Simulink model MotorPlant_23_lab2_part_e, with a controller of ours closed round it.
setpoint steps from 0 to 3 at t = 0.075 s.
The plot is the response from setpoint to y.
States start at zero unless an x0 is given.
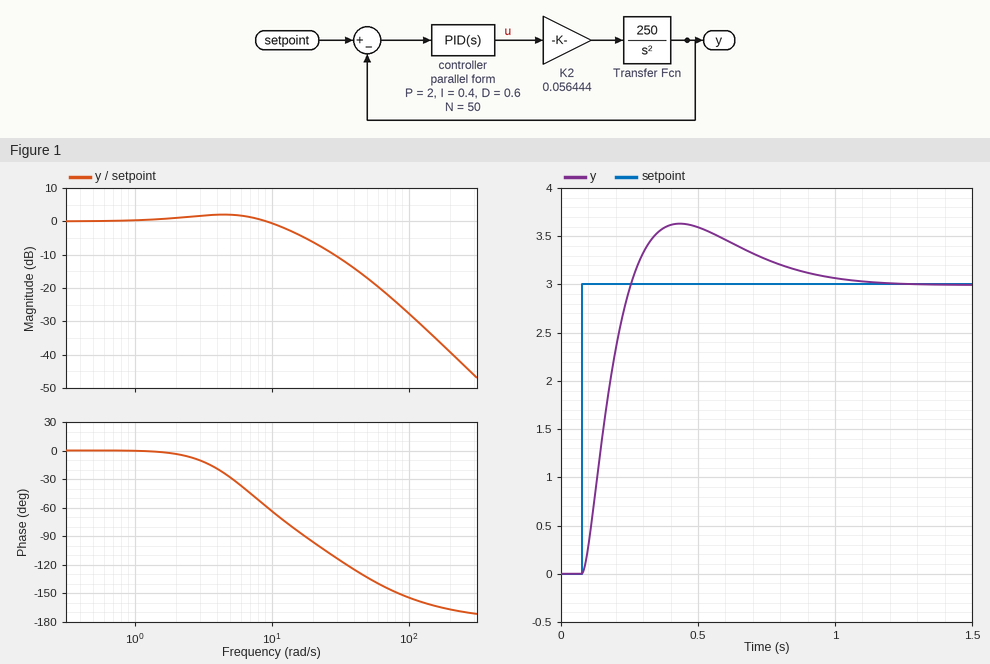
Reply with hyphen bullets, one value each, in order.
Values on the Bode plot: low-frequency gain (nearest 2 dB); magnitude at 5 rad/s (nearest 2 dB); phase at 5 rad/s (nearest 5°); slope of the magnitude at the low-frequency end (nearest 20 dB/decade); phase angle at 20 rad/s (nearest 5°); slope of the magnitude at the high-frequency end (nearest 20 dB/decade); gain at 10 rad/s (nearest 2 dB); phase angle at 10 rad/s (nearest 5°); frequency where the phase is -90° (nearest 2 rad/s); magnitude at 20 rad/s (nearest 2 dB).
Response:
- 0 dB
- 2 dB
- -30°
- 0 dB/decade
- -95°
- -40 dB/decade
- 0 dB
- -65°
- 18 rad/s
- -6 dB
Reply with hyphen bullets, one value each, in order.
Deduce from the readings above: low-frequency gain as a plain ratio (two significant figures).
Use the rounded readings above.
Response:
- 1.0
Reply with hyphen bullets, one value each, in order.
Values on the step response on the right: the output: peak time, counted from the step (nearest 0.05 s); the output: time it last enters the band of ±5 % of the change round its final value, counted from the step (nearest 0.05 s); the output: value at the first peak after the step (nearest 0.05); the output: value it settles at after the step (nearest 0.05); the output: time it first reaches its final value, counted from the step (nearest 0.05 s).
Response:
- 0.35 s
- 0.80 s
- 3.65
- 3.00
- 0.20 s
